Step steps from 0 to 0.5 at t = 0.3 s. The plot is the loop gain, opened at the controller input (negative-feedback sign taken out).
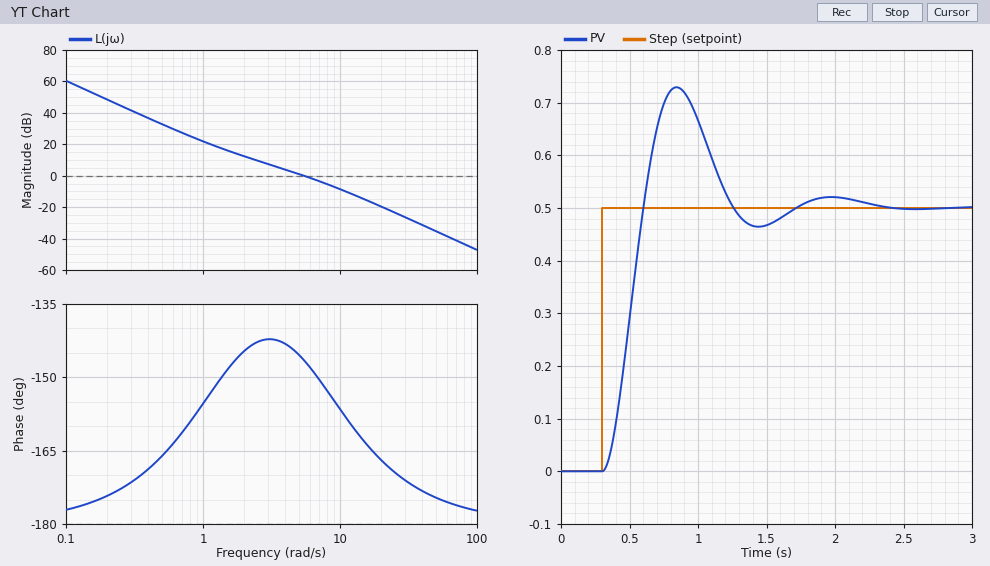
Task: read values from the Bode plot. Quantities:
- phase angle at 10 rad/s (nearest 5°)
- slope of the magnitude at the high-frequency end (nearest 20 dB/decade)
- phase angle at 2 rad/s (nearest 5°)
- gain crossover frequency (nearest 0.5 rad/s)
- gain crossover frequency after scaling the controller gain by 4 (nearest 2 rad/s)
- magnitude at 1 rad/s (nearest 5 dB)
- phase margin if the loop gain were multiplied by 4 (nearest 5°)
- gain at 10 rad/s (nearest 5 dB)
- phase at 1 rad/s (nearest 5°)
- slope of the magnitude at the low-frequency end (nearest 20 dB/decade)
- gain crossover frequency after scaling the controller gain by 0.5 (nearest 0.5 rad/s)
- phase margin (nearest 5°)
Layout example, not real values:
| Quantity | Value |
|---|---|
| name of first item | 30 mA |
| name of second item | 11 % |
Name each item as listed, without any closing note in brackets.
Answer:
| Quantity | Value |
|---|---|
| phase angle at 10 rad/s | -155° |
| slope of the magnitude at the high-frequency end | -40 dB/decade |
| phase angle at 2 rad/s | -145° |
| gain crossover frequency | 5.5 rad/s |
| gain crossover frequency after scaling the controller gain by 4 | 12 rad/s |
| magnitude at 1 rad/s | 20 dB |
| phase margin if the loop gain were multiplied by 4 | 20° |
| gain at 10 rad/s | -10 dB |
| phase at 1 rad/s | -155° |
| slope of the magnitude at the low-frequency end | -40 dB/decade |
| gain crossover frequency after scaling the controller gain by 0.5 | 3.5 rad/s |
| phase margin | 35° |
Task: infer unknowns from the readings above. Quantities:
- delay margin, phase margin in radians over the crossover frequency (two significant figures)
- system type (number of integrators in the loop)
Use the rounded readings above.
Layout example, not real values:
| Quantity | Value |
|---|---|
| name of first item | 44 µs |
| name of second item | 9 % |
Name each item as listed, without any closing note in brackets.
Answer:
| Quantity | Value |
|---|---|
| delay margin, phase margin in radians over the crossover frequency | 0.11 s |
| system type | 2 |
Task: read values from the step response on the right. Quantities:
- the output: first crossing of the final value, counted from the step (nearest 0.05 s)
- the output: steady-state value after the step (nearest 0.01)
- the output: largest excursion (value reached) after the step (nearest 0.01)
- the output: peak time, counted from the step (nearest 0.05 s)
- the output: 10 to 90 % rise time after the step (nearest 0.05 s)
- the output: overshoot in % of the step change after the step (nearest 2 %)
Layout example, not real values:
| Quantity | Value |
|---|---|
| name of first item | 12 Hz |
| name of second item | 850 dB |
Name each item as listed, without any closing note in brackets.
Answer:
| Quantity | Value |
|---|---|
| the output: first crossing of the final value, counted from the step | 0.30 s |
| the output: steady-state value after the step | 0.50 |
| the output: largest excursion (value reached) after the step | 0.73 |
| the output: peak time, counted from the step | 0.55 s |
| the output: 10 to 90 % rise time after the step | 0.20 s |
| the output: overshoot in % of the step change after the step | 46 % |
